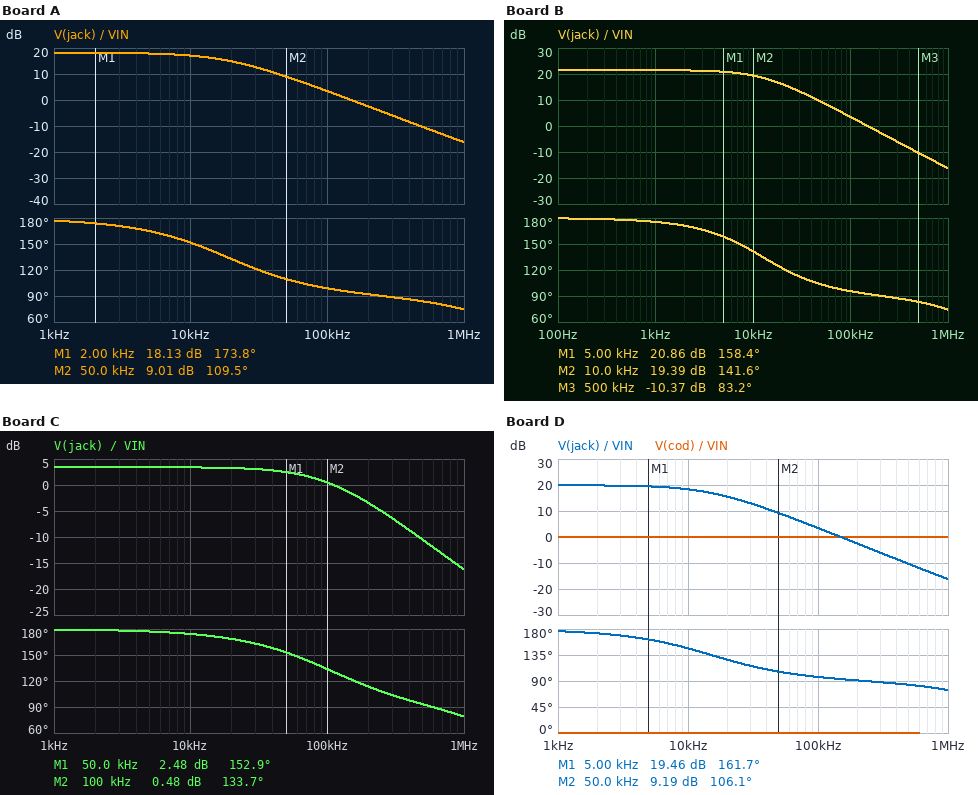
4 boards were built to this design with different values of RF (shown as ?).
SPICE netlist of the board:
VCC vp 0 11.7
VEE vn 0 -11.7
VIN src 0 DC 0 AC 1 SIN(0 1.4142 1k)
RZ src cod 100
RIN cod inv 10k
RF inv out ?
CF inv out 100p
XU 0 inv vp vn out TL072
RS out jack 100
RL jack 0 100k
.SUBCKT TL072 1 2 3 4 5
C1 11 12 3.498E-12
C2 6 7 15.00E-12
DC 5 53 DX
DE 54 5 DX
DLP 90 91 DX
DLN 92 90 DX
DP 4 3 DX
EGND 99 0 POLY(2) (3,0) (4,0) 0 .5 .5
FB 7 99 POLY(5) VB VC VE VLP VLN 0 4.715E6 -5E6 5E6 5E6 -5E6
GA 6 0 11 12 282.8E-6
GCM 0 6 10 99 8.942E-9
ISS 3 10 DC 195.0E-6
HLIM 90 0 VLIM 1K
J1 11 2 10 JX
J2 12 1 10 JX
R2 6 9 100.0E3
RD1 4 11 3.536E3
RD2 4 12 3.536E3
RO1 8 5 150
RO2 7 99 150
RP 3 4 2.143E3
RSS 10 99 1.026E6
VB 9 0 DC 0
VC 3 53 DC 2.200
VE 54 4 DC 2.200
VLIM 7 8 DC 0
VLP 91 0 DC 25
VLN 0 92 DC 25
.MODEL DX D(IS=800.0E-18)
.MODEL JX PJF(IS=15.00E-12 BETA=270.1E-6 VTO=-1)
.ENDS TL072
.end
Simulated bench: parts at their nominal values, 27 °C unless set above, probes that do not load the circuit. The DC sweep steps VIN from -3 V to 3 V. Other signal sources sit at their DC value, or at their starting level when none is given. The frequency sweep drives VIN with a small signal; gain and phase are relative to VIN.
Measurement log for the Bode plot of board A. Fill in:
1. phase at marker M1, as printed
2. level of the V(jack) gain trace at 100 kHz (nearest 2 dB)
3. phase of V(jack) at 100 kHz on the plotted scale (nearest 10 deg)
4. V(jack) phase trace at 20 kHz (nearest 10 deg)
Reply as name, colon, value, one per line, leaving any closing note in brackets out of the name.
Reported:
phase at marker M1, as printed: 173.8 deg
level of the V(jack) gain trace at 100 kHz: 4 dB
phase of V(jack) at 100 kHz on the plotted scale: 100 deg
V(jack) phase trace at 20 kHz: 130 deg
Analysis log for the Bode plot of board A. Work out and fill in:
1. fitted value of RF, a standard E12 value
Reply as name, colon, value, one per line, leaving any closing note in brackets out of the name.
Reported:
fitted value of RF, a standard E12 value: 82 kΩ
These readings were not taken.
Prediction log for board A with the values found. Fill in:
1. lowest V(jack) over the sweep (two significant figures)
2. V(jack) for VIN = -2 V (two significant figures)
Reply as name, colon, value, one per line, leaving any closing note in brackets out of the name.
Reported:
lowest V(jack) over the sweep: -10 V
V(jack) for VIN = -2 V: 10 V
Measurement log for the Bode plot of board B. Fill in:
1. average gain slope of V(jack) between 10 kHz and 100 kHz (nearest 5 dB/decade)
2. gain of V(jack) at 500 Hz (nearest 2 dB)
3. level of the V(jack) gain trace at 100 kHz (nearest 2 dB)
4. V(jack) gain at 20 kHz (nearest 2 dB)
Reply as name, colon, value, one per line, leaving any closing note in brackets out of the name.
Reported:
average gain slope of V(jack) between 10 kHz and 100 kHz: -15 dB/decade
gain of V(jack) at 500 Hz: 22 dB
level of the V(jack) gain trace at 100 kHz: 4 dB
V(jack) gain at 20 kHz: 16 dB
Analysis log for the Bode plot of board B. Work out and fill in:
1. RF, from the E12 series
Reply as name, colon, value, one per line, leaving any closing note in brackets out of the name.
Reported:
RF, from the E12 series: 120 kΩ
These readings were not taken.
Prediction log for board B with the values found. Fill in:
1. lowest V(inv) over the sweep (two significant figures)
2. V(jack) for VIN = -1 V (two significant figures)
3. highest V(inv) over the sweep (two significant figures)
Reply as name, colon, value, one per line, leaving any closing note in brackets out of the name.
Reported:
lowest V(inv) over the sweep: -2.0 V
V(jack) for VIN = -1 V: 10 V
highest V(inv) over the sweep: 2.0 V
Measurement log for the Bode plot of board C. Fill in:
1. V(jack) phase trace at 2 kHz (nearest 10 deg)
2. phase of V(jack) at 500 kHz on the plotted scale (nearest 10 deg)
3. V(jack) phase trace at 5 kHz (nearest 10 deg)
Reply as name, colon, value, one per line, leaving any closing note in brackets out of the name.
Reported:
V(jack) phase trace at 2 kHz: 180 deg
phase of V(jack) at 500 kHz on the plotted scale: 90 deg
V(jack) phase trace at 5 kHz: 180 deg
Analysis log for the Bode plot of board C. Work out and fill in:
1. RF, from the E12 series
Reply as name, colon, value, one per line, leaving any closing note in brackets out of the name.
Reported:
RF, from the E12 series: 15 kΩ
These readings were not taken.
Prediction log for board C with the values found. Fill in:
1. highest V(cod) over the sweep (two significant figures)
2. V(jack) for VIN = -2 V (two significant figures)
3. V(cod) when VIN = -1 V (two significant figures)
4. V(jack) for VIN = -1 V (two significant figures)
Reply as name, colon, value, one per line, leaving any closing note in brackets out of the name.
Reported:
highest V(cod) over the sweep: 3.0 V
V(jack) for VIN = -2 V: 3.0 V
V(cod) when VIN = -1 V: -990 mV
V(jack) for VIN = -1 V: 1.5 V
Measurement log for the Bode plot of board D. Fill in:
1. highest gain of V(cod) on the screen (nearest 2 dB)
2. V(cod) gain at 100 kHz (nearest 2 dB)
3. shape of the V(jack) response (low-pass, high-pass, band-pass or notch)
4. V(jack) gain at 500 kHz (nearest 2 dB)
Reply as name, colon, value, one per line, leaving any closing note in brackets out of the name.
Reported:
highest gain of V(cod) on the screen: 0 dB
V(cod) gain at 100 kHz: 0 dB
shape of the V(jack) response: low-pass
V(jack) gain at 500 kHz: -10 dB
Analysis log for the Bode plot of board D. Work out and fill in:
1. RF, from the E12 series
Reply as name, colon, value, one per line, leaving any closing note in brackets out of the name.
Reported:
RF, from the E12 series: 100 kΩ
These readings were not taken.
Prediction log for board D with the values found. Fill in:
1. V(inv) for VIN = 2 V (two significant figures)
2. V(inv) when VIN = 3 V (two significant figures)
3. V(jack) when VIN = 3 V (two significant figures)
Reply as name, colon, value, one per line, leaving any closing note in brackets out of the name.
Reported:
V(inv) for VIN = 2 V: 880 mV
V(inv) when VIN = 3 V: 1.8 V
V(jack) when VIN = 3 V: -10 V
